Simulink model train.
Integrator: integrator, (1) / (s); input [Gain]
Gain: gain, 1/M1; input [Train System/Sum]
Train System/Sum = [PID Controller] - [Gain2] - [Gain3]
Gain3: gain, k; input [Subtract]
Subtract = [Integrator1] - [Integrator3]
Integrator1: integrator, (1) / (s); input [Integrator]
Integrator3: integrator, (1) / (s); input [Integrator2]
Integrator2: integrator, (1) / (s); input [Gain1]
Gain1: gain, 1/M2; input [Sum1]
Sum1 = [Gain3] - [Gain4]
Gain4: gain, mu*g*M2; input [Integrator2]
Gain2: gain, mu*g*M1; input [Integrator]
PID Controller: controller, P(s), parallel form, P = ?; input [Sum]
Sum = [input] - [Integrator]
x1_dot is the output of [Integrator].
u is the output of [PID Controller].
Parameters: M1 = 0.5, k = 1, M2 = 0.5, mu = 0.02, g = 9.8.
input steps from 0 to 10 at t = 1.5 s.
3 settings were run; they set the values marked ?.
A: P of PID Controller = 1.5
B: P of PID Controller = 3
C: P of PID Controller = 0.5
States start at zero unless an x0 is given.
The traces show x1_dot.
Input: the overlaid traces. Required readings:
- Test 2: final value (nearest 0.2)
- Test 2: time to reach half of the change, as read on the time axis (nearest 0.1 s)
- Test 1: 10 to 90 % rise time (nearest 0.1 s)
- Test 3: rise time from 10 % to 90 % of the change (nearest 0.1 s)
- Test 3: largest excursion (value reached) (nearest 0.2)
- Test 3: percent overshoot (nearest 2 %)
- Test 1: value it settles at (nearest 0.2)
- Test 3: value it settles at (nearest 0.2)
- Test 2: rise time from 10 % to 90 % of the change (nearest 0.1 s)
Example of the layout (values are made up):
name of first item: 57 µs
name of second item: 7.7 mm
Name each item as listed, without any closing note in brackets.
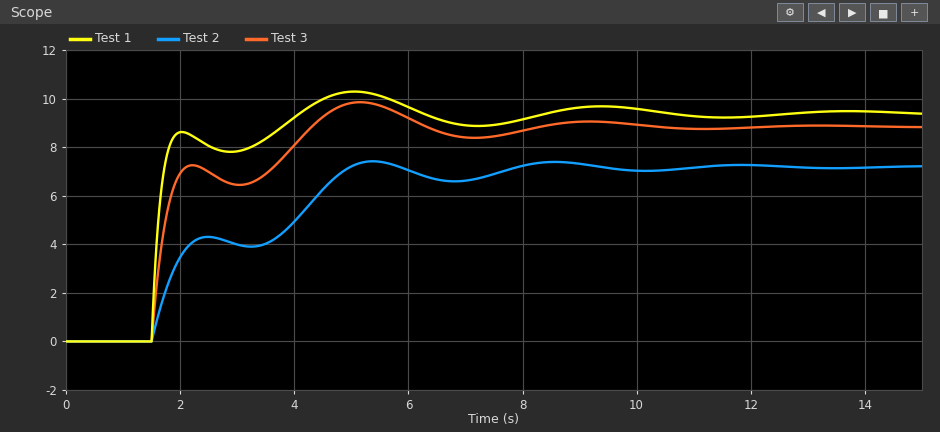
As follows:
Test 2: final value: 7.2
Test 2: time to reach half of the change, as read on the time axis: 2.0 s
Test 1: 10 to 90 % rise time: 0.4 s
Test 3: rise time from 10 % to 90 % of the change: 2.4 s
Test 3: largest excursion (value reached): 9.8
Test 3: percent overshoot: 12 %
Test 1: value it settles at: 9.4
Test 3: value it settles at: 8.8
Test 2: rise time from 10 % to 90 % of the change: 3.0 s
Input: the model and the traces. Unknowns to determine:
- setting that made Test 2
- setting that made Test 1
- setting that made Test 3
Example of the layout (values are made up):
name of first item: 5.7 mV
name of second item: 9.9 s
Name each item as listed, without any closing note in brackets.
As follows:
setting that made Test 2: C
setting that made Test 1: B
setting that made Test 3: A
